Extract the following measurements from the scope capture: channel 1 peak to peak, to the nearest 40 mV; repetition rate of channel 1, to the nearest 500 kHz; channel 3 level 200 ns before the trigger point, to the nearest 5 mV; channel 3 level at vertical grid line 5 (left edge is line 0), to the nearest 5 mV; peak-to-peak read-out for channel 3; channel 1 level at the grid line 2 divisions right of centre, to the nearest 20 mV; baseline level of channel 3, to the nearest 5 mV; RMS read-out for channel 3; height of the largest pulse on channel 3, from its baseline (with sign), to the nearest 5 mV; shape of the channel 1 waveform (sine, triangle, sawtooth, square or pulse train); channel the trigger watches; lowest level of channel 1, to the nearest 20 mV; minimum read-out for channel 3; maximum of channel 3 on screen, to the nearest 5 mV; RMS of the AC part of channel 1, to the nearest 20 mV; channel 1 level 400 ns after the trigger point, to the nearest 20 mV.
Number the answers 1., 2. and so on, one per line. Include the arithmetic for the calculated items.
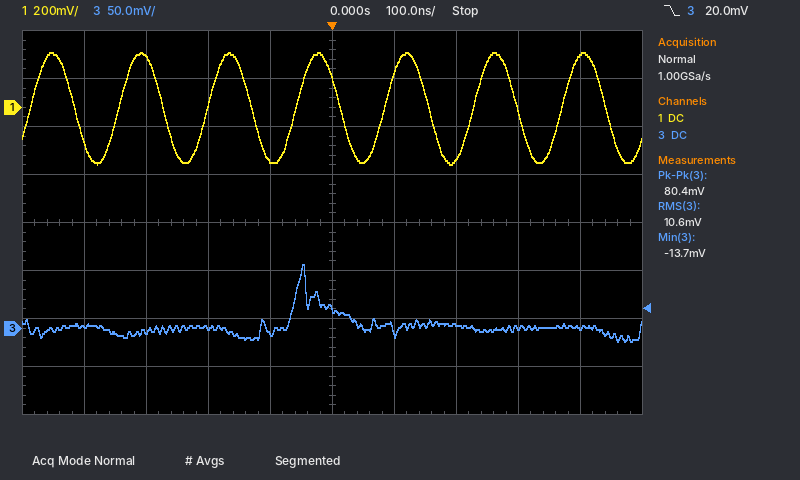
1. 480 mV
2. 7.0 MHz
3. 0 mV
4. 20 mV
5. 80.4 mV
6. -220 mV
7. 0 mV
8. 10.6 mV
9. 65 mV − (0 mV) = +65 mV
10. sine
11. channel 3
12. -240 mV
13. -13.7 mV
14. 65 mV
15. 480 mV / (2√2) ≈ 170 mV, so 160 mV to the nearest 20 mV
16. 220 mV
